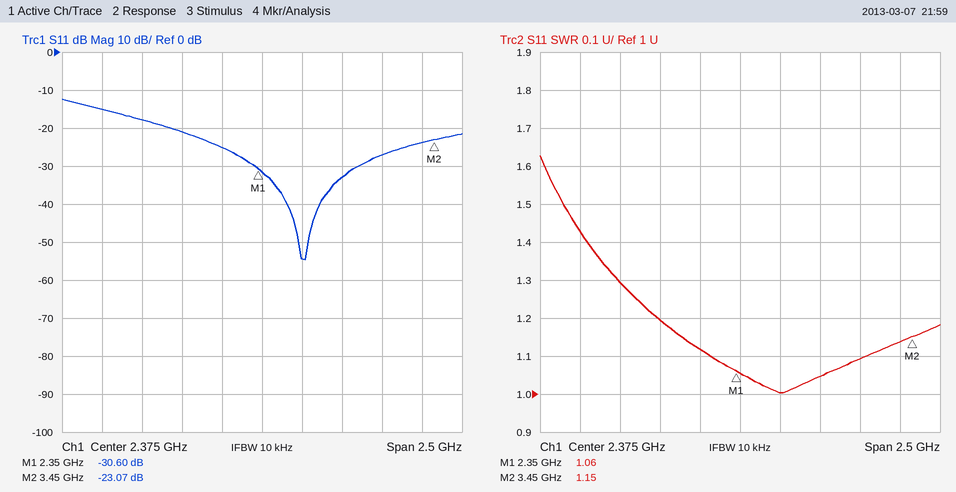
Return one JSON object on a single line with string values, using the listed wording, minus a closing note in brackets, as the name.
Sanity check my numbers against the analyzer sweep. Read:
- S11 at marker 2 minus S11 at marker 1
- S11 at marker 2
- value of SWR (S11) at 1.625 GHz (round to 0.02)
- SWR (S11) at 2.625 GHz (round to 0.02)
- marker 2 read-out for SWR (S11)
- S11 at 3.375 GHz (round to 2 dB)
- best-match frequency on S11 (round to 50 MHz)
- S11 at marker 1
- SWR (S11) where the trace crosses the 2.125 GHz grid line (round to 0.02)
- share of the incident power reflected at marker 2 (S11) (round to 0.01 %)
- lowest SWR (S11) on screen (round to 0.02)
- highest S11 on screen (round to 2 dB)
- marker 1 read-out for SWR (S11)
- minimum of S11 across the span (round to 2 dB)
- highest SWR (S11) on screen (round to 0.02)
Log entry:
{"S11 at marker 2 minus S11 at marker 1": "7.53 dB", "S11 at marker 2": "-23.07 dB", "value of SWR (S11) at 1.625 GHz": "1.30", "SWR (S11) at 2.625 GHz": "1.00", "marker 2 read-out for SWR": "1.15", "S11 at 3.375 GHz": "-24 dB", "best-match frequency on S11": "2.65 GHz", "S11 at marker 1": "-30.60 dB", "SWR (S11) where the trace crosses the 2.125 GHz grid line": "1.12", "share of the incident power reflected at marker 2 (S11)": "0.49 %", "lowest SWR (S11) on screen": "1.00", "highest S11 on screen": "-12 dB", "marker 1 read-out for SWR": "1.06", "minimum of S11 across the span": "-54 dB", "highest SWR (S11) on screen": "1.62"}
